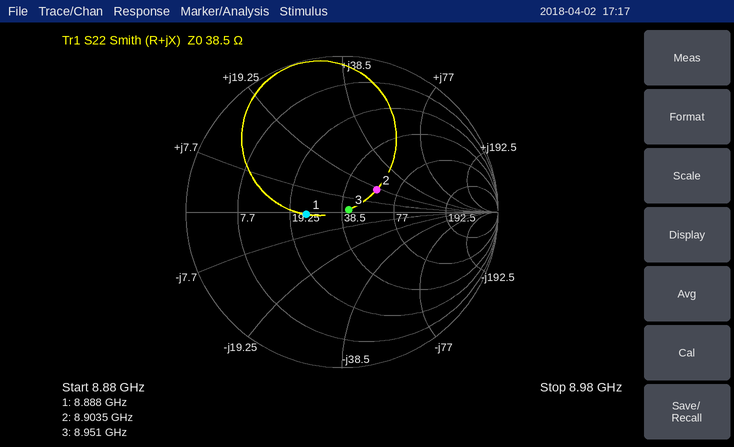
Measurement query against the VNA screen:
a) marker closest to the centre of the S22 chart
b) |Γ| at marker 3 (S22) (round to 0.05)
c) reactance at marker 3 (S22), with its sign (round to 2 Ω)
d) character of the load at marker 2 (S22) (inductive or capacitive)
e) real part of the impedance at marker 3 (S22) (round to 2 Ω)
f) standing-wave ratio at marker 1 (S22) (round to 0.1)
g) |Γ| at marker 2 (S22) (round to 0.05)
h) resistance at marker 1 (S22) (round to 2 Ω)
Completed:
marker 3
0.05
+2 Ω
inductive
42 Ω
1.6
0.25
24 Ω
